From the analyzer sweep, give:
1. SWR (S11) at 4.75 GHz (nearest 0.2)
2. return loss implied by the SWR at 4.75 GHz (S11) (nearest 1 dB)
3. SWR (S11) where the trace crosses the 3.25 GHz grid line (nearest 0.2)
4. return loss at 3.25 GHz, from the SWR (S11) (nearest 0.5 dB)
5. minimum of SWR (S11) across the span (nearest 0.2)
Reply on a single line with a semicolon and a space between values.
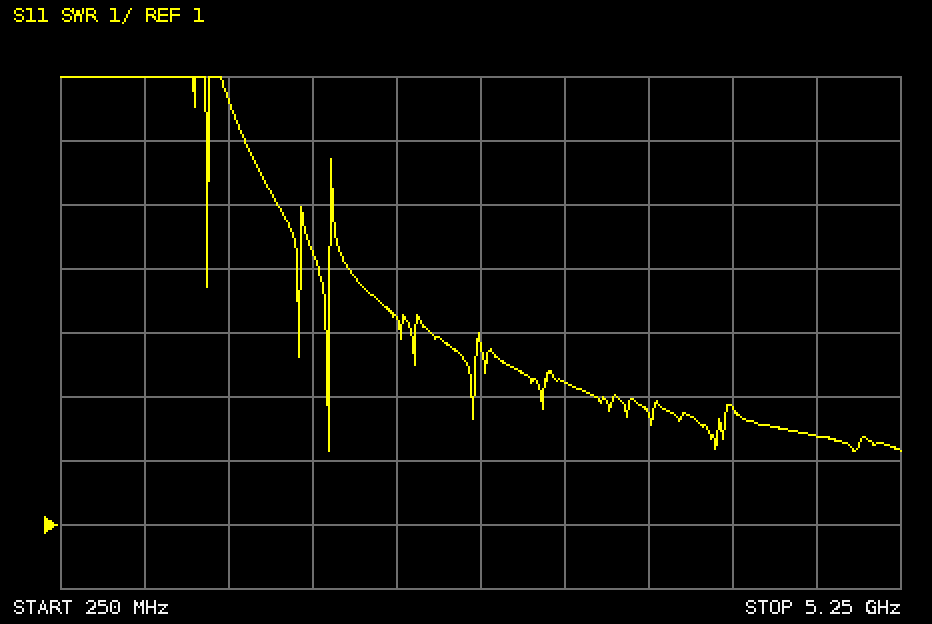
2.4; 8 dB; 3.2; 5.5 dB; 2.2
